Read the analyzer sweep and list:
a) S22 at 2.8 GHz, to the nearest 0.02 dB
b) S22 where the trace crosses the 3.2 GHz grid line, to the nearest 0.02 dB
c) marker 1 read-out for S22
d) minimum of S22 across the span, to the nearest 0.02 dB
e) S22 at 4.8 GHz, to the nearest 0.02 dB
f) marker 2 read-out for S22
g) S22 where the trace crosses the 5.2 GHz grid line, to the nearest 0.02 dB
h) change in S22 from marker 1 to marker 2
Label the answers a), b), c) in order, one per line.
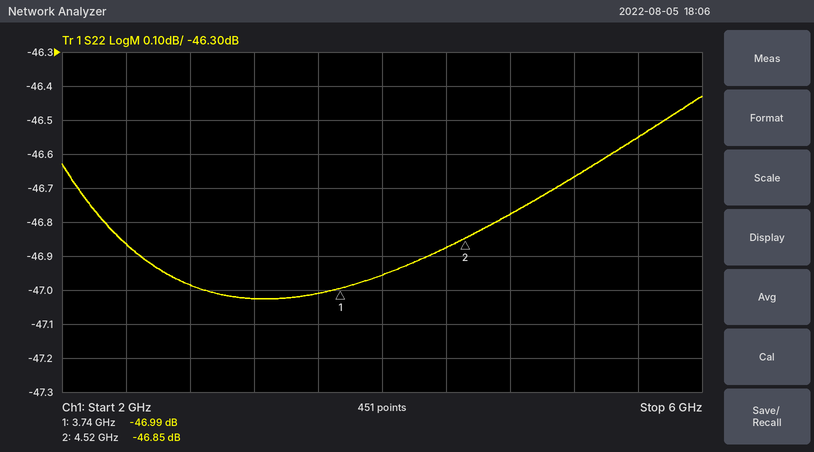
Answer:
a) -46.98 dB
b) -47.02 dB
c) -46.99 dB
d) -47.02 dB
e) -46.78 dB
f) -46.85 dB
g) -46.66 dB
h) 0.14 dB
